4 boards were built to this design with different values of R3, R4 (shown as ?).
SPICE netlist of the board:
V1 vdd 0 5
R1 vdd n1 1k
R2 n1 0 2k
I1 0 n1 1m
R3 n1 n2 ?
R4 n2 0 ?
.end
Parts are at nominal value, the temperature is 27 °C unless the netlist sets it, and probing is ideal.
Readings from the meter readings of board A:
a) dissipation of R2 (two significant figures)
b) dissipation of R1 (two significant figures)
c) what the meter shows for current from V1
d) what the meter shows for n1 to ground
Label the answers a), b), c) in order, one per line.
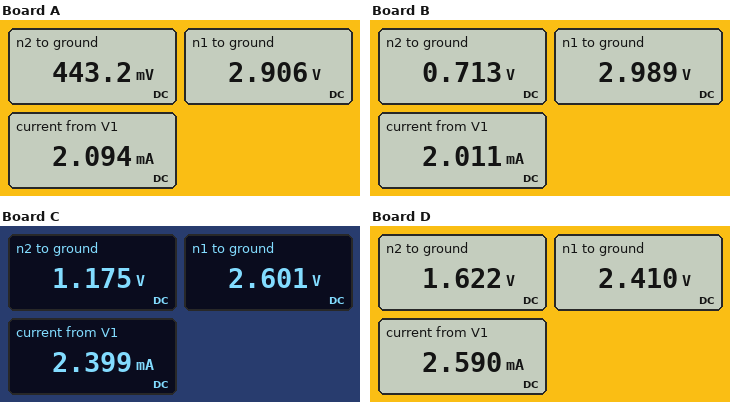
a) 4.2 mW
b) 4.4 mW
c) 2.094 mA
d) 2.906 V
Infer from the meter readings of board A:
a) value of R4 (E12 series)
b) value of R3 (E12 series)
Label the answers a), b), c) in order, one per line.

a) 270 Ω
b) 1.5 kΩ
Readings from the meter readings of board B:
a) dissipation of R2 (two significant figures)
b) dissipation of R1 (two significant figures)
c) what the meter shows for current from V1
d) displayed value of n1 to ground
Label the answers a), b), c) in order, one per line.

a) 4.5 mW
b) 4.0 mW
c) 2.011 mA
d) 2.989 V
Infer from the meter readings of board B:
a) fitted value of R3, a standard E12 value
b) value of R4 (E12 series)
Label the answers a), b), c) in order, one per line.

a) 1.5 kΩ
b) 470 Ω
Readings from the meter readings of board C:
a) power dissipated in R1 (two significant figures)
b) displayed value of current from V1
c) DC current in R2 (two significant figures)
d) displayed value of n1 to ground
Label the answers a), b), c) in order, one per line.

a) 5.8 mW
b) 2.399 mA
c) 1.3 mA
d) 2.601 V
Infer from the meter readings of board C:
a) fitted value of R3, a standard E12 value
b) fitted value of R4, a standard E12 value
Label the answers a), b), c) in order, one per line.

a) 680 Ω
b) 560 Ω
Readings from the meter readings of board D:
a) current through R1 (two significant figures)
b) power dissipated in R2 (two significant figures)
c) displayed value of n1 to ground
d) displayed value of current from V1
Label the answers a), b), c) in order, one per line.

a) 2.6 mA
b) 2.9 mW
c) 2.410 V
d) 2.590 mA
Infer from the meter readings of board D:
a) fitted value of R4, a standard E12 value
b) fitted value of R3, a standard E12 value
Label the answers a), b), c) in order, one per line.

a) 680 Ω
b) 330 Ω
